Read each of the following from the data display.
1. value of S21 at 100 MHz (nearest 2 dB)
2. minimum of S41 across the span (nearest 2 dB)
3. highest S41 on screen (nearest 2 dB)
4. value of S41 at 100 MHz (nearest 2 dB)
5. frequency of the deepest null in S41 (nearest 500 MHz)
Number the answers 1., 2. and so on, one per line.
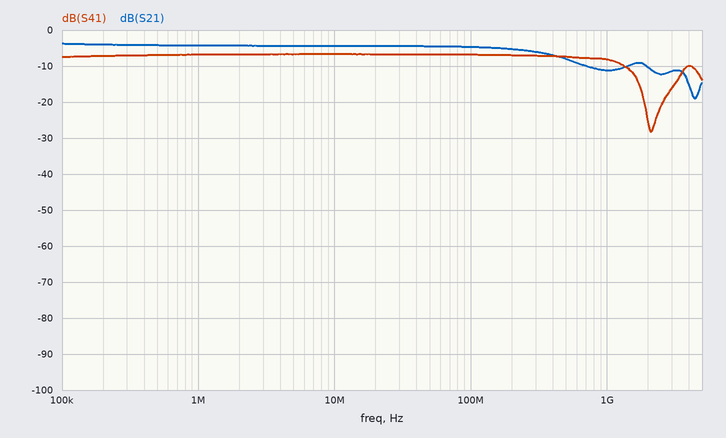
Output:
1. -4 dB
2. -28 dB
3. -6 dB
4. -6 dB
5. 2.0 GHz
